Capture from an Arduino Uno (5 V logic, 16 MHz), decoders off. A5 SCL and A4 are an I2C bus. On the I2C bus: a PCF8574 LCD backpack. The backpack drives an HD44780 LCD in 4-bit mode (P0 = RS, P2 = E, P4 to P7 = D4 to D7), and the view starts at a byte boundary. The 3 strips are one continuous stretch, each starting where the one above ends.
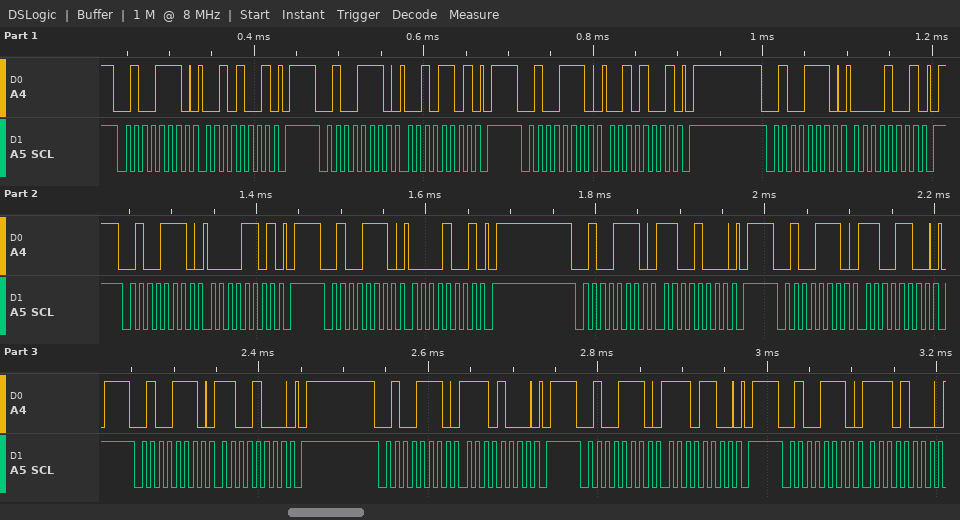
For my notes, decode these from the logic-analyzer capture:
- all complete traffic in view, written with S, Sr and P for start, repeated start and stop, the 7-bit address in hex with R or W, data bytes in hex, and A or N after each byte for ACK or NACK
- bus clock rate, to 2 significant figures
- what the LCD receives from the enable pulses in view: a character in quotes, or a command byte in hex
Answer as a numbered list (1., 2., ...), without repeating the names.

1. S 27W A 29 A P S 27W A 2D A P S 27W A 29 A P S 27W A 09 A P S 27W A 0D A P S 27W A 09 A P S 27W A C8 A P S 27W A CC A P S 27W A C8 A P S 27W A E8 A P S 27W A EC A P S 27W A E8 A
2. 100 kHz
3. ' ' 0xCE
